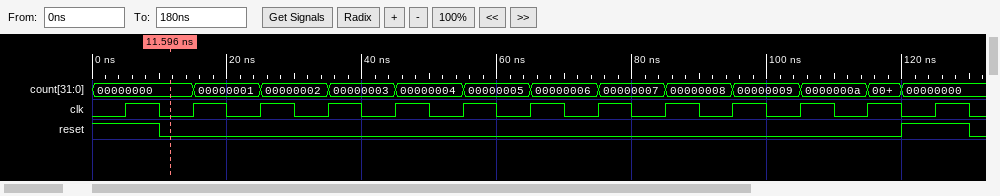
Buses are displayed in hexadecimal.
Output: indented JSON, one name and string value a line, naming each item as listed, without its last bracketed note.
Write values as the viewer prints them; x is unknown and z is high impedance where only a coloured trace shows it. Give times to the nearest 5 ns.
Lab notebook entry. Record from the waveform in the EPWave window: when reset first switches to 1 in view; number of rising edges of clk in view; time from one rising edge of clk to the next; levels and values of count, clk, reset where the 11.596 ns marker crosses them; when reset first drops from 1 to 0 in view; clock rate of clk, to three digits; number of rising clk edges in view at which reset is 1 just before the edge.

{
  "when reset first switches to 1 in view": "120 ns",
  "number of rising edges of clk in view": "13",
  "time from one rising edge of clk to the next": "10 ns",
  "levels and values of count, clk, reset where the 11.596 ns marker crosses them": "count=00000000, clk=0, reset=0",
  "when reset first drops from 1 to 0 in view": "10 ns",
  "clock rate of clk, to three digits": "100 MHz",
  "number of rising clk edges in view at which reset is 1 just before the edge": "2"
}
